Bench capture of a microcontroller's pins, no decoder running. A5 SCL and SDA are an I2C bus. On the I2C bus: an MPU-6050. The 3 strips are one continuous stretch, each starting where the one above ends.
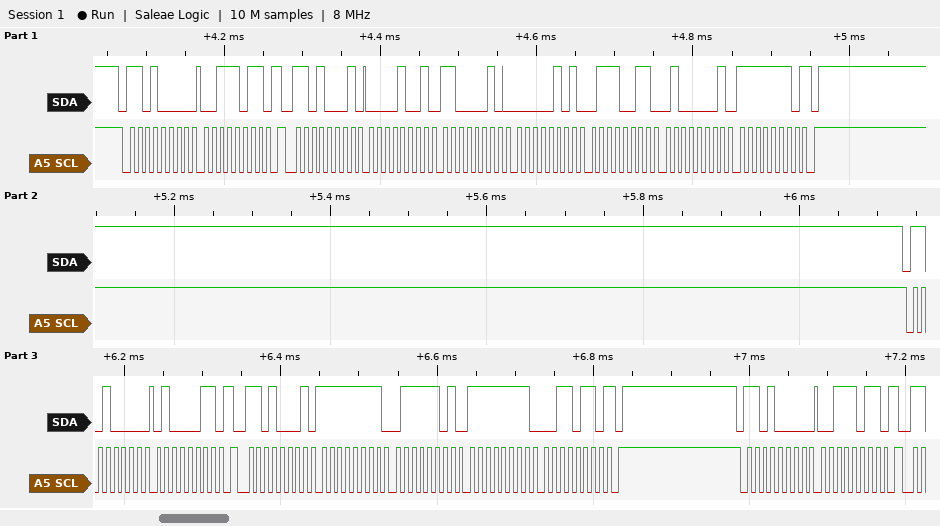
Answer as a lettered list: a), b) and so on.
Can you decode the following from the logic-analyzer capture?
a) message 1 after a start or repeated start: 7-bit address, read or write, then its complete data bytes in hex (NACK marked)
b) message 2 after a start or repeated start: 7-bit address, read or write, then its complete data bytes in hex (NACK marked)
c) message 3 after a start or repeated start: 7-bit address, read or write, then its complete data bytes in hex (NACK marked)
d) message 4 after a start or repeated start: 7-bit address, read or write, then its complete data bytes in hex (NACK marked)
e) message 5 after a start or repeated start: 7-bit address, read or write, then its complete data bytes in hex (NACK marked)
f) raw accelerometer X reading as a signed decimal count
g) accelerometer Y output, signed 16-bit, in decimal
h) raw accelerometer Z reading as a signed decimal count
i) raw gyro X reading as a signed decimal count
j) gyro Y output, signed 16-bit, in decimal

a) 0x68 write: 3B
b) 0x68 read: 09 C2 05 73 41 FE NACK
c) 0x68 write: 43
d) 0x68 read: FF 7D FF 36 NACK
e) 0x68 write: 3B
f) 2498
g) 1395
h) 16894
i) -131
j) -202
